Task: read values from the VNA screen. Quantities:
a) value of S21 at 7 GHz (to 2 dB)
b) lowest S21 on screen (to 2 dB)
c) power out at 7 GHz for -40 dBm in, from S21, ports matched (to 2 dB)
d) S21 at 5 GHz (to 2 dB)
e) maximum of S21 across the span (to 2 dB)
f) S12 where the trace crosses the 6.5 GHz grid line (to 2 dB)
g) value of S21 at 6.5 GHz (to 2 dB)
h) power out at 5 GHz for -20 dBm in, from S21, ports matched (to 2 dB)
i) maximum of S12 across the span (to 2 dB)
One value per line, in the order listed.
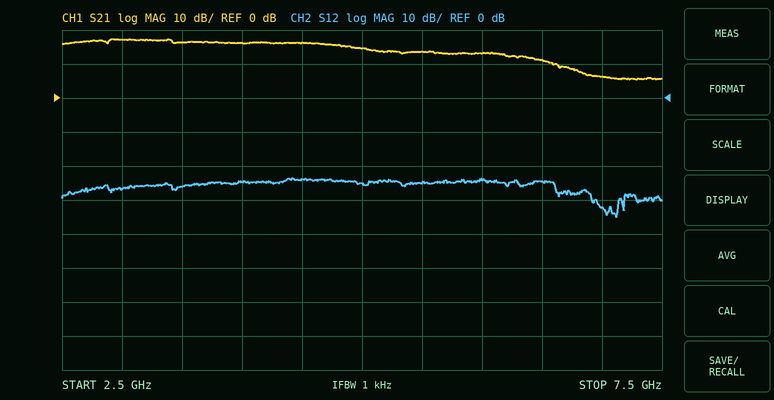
6 dB
6 dB
-34 dBm
14 dB
18 dB
-24 dB
12 dB
-6 dBm
-24 dB
